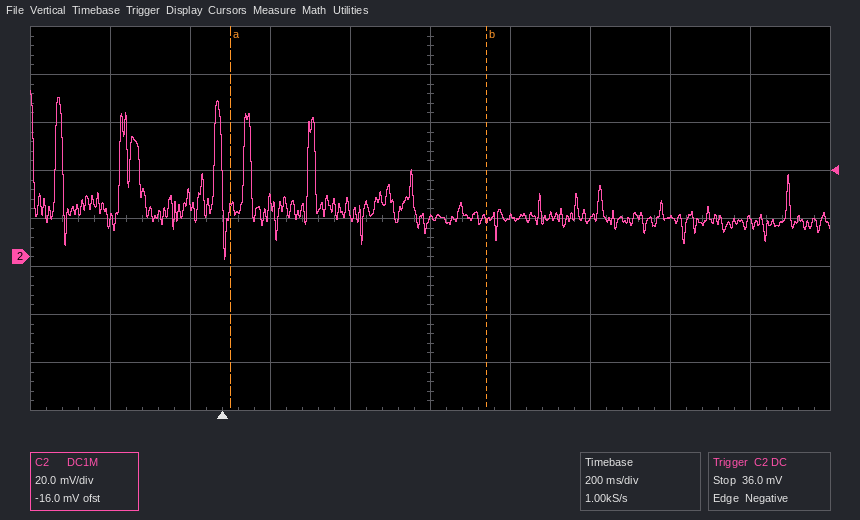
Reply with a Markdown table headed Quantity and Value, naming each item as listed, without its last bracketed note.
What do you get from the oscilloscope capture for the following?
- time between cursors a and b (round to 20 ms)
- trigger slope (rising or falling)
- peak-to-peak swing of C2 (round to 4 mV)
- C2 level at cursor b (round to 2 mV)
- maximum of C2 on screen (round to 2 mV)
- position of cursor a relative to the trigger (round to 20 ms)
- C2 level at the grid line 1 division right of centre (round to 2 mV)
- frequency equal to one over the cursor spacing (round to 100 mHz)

| Quantity | Value |
|---|---|
| time between cursors a and b | 640 ms |
| trigger slope | falling |
| peak-to-peak swing of C2 | 72 mV |
| C2 level at cursor b | 16 mV |
| maximum of C2 on screen | 70 mV |
| position of cursor a relative to the trigger | +20 ms |
| C2 level at the grid line 1 division right of centre | 16 mV |
| frequency equal to one over the cursor spacing | 1.6 Hz |
